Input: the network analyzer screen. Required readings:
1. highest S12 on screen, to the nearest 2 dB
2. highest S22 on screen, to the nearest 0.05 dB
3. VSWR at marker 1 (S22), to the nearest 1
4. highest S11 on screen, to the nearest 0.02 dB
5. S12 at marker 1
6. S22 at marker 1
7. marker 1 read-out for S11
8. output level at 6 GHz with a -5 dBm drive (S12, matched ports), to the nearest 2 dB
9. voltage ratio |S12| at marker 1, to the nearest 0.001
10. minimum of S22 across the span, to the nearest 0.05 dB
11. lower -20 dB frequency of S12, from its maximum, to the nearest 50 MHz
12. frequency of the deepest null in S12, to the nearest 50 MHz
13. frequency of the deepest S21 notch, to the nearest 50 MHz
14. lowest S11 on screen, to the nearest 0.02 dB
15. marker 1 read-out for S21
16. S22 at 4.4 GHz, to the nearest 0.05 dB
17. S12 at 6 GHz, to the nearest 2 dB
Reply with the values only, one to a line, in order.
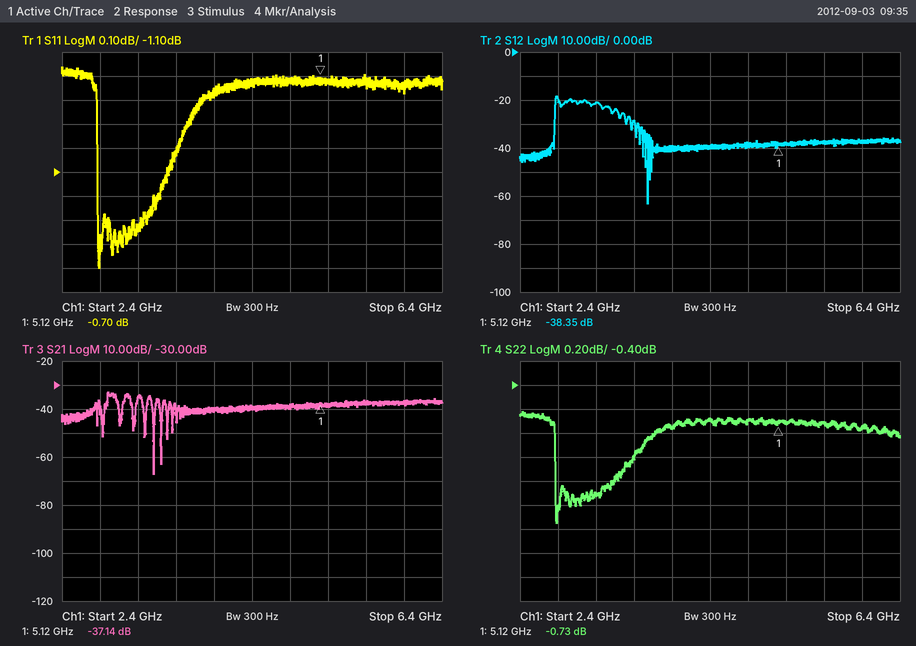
-18 dB
-0.60 dB
24
-0.66 dB
-38.35 dB
-0.73 dB
-0.70 dB
-42 dBm
0.012
-1.55 dB
2.75 GHz
3.75 GHz
3.35 GHz
-1.50 dB
-37.14 dB
-0.70 dB
-38 dB
